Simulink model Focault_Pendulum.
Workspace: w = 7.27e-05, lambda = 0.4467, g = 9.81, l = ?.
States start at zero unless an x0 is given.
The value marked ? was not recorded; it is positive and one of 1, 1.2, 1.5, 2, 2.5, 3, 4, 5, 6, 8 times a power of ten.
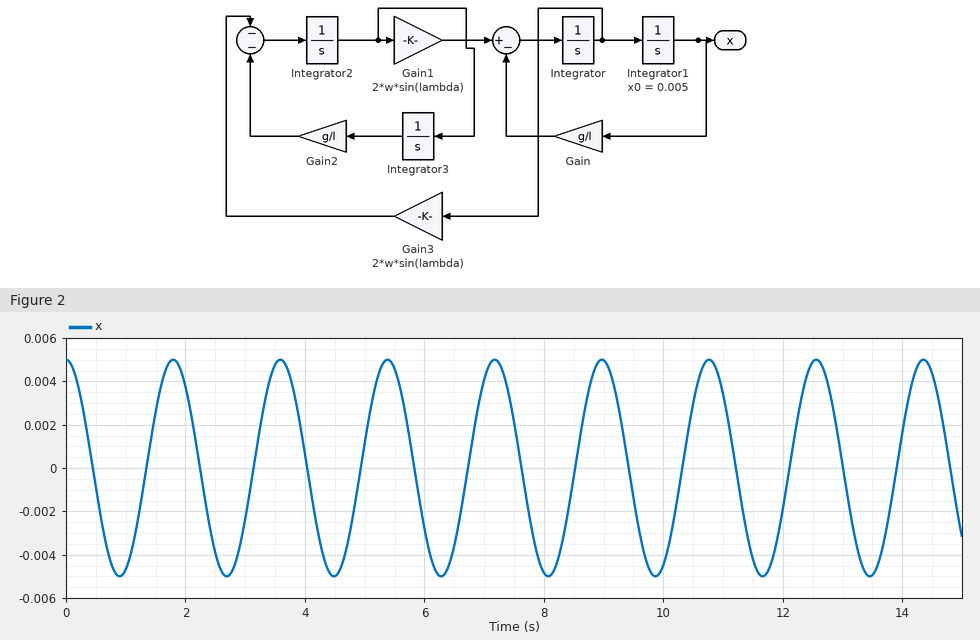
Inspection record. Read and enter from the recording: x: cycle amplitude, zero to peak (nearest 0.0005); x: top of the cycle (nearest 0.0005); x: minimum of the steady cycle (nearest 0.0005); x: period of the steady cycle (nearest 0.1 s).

0.0050
0.0050
-0.0050
1.8 s
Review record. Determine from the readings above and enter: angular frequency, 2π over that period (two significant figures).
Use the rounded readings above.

3.5 rad/s
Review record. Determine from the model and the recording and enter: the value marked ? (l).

0.8
